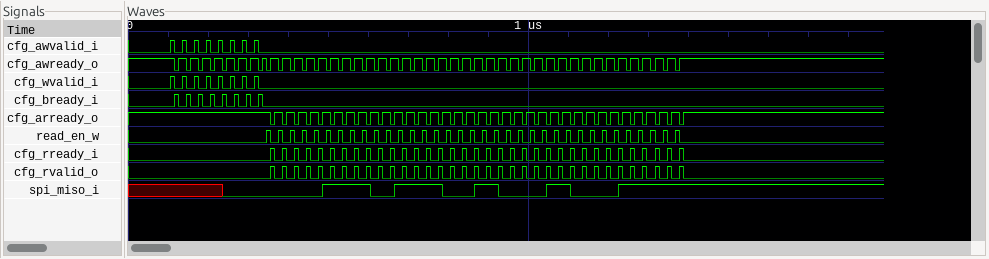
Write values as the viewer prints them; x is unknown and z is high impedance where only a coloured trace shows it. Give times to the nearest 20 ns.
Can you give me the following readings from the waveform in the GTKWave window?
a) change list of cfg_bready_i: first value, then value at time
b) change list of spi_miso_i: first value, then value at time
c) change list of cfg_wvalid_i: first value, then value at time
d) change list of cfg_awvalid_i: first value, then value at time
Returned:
0, 1 at 120 ns, 0 at 120 ns, 1 at 140 ns, 0 at 160 ns, 1 at 180 ns, 0 at 180 ns, 1 at 200 ns, 0 at 220 ns, 1 at 240 ns, 0 at 240 ns, 1 at 260 ns, 0 at 280 ns, 1 at 300 ns, 0 at 300 ns, 1 at 320 ns, 0 at 340 ns
x, 0 at 240 ns, 1 at 480 ns, 0 at 600 ns, 1 at 660 ns, 0 at 780 ns, 1 at 860 ns, 0 at 920 ns, 1 at 1040 ns, 0 at 1100 ns, 1 at 1220 ns
0, 1 at 100 ns, 0 at 120 ns, 1 at 140 ns, 0 at 140 ns, 1 at 160 ns, 0 at 180 ns, 1 at 200 ns, 0 at 200 ns, 1 at 220 ns, 0 at 240 ns, 1 at 260 ns, 0 at 260 ns, 1 at 280 ns, 0 at 300 ns, 1 at 320 ns, 0 at 320 ns
0, 1 at 100 ns, 0 at 120 ns, 1 at 140 ns, 0 at 140 ns, 1 at 160 ns, 0 at 180 ns, 1 at 200 ns, 0 at 200 ns, 1 at 220 ns, 0 at 240 ns, 1 at 260 ns, 0 at 260 ns, 1 at 280 ns, 0 at 300 ns, 1 at 320 ns, 0 at 320 ns
